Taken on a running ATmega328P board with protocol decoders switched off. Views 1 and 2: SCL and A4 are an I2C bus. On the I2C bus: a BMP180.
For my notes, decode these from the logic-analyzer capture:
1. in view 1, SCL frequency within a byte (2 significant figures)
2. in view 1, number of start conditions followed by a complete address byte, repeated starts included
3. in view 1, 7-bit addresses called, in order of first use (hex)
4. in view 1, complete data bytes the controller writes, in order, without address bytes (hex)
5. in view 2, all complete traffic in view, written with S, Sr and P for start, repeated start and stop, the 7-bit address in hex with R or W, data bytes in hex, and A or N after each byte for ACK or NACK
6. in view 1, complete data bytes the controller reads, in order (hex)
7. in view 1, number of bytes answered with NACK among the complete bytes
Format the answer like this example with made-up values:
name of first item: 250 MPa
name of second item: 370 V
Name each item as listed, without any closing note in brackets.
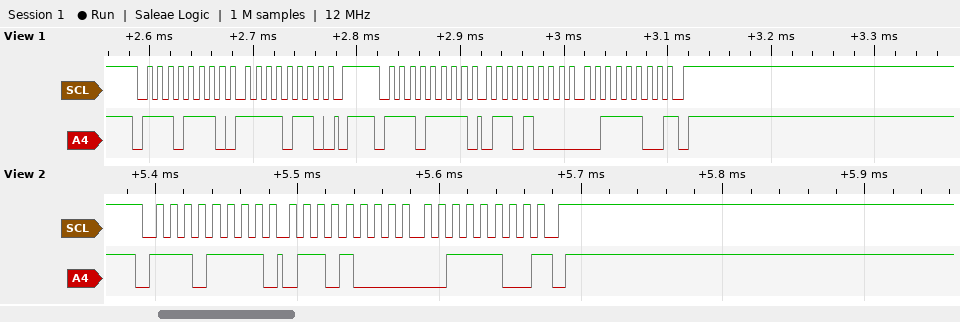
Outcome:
in view 1, SCL frequency within a byte: 100 kHz
in view 1, number of start conditions followed by a complete address byte, repeated starts included: 2
in view 1, 7-bit addresses called, in order of first use: 0x77
in view 1, complete data bytes the controller writes, in order, without address bytes: F6
in view 2, all complete traffic in view, written with S, Sr and P for start, repeated start and stop, the 7-bit address in hex with R or W, data bytes in hex, and A or N after each byte for ACK or NACK: S 77R A 68 A 3C N P
in view 1, complete data bytes the controller reads, in order: 68 3C
in view 1, number of bytes answered with NACK among the complete bytes: 1
